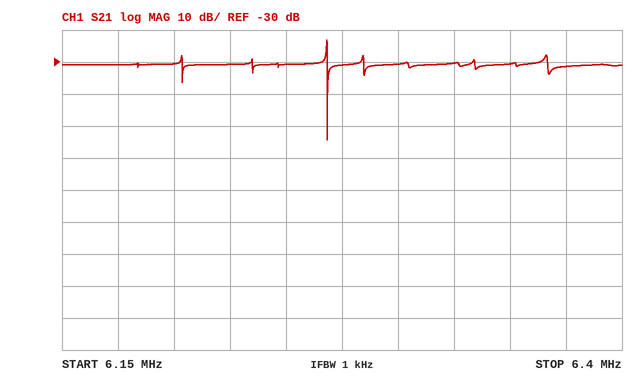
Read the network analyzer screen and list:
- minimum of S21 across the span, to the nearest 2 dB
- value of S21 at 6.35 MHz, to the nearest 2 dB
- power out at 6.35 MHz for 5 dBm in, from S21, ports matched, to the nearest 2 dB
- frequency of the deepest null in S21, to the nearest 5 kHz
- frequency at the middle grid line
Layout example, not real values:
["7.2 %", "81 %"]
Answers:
["-54 dB", "-30 dB", "-26 dBm", "6.270 MHz", "6.275 MHz"]
